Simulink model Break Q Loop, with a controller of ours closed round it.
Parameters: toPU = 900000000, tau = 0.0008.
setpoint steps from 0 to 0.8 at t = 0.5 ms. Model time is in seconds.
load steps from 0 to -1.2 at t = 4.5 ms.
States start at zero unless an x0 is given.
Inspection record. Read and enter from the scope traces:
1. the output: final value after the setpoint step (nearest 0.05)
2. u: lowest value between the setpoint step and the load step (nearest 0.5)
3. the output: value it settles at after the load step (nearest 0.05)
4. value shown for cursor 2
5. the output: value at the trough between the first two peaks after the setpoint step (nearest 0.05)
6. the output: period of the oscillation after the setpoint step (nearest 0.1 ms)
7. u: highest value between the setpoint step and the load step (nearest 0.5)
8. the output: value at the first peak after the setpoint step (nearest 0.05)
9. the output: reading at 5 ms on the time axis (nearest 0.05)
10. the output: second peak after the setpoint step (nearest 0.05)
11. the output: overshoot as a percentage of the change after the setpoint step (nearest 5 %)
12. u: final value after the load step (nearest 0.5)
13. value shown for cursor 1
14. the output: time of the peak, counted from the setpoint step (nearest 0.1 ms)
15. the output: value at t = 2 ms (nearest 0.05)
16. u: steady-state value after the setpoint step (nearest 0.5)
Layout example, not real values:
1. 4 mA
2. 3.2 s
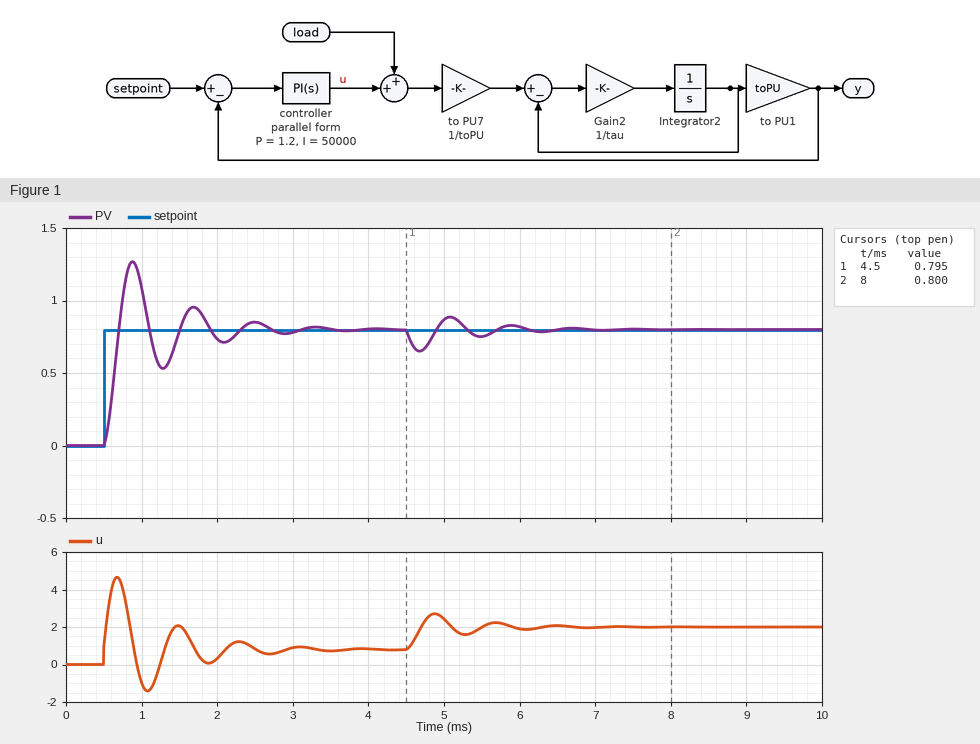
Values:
1. 0.80
2. -1.5
3. 0.80
4. 0.800
5. 0.55
6. 0.8 ms
7. 4.5
8. 1.25
9. 0.85
10. 0.95
11. 60 %
12. 2.0
13. 0.795
14. 0.4 ms
15. 0.75
16. 1.0
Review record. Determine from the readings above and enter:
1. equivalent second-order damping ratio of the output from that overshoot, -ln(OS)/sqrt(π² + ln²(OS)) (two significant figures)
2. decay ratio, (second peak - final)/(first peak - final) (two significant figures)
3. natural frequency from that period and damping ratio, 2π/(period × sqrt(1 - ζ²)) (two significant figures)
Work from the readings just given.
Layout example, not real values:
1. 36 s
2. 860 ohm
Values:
1. 0.16
2. 0.33
3. 8.0 rad/ms
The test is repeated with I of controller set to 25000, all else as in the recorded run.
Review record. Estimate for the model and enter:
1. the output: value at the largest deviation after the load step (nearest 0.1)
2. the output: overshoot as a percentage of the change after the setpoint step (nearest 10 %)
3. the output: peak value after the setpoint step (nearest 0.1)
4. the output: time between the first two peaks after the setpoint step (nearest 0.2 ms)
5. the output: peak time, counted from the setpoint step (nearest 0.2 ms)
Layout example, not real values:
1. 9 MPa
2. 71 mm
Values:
1. 0.6
2. 50 %
3. 1.2
4. 1.2 ms
5. 0.6 ms
